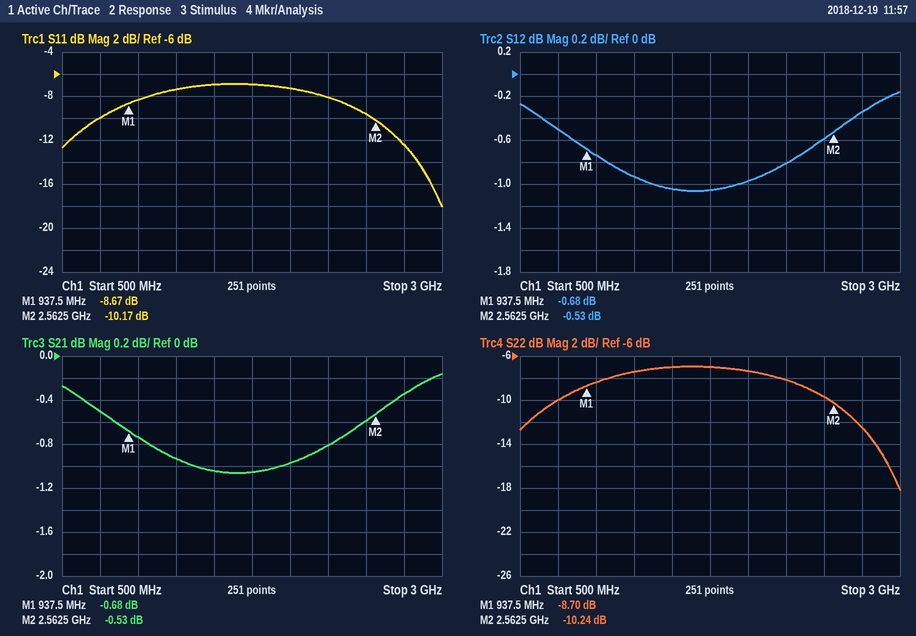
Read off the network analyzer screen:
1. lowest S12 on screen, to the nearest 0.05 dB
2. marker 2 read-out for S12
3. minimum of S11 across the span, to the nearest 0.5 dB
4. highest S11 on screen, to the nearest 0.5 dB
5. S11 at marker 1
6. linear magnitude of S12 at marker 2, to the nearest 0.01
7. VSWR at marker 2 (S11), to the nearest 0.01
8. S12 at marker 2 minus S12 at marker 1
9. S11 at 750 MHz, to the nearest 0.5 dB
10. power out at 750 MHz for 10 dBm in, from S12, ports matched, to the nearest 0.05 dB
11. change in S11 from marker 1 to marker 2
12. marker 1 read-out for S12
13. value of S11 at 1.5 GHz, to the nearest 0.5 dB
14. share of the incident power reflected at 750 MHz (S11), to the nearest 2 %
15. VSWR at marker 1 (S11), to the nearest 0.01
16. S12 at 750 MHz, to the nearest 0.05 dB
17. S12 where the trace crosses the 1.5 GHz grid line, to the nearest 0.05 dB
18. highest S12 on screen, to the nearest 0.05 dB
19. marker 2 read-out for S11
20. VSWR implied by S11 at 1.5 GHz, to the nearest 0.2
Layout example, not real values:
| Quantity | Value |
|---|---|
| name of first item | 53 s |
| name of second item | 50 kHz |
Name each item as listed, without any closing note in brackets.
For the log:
| Quantity | Value |
|---|---|
| lowest S12 on screen, to the nearest 0.05 dB | -1.05 dB |
| marker 2 read-out for S12 | -0.53 dB |
| minimum of S11 across the span, to the nearest 0.5 dB | -18.0 dB |
| highest S11 on screen, to the nearest 0.5 dB | -7.0 dB |
| S11 at marker 1 | -8.67 dB |
| linear magnitude of S12 at marker 2, to the nearest 0.01 | 0.94 |
| VSWR at marker 2 (S11), to the nearest 0.01 | 1.90 |
| S12 at marker 2 minus S12 at marker 1 | 0.15 dB |
| S11 at 750 MHz, to the nearest 0.5 dB | -10.0 dB |
| power out at 750 MHz for 10 dBm in, from S12, ports matched, to the nearest 0.05 dB | 9.50 dBm |
| change in S11 from marker 1 to marker 2 | -1.50 dB |
| marker 1 read-out for S12 | -0.68 dB |
| value of S11 at 1.5 GHz, to the nearest 0.5 dB | -7.0 dB |
| share of the incident power reflected at 750 MHz (S11), to the nearest 2 % | 10 % |
| VSWR at marker 1 (S11), to the nearest 0.01 | 2.17 |
| S12 at 750 MHz, to the nearest 0.05 dB | -0.50 dB |
| S12 where the trace crosses the 1.5 GHz grid line, to the nearest 0.05 dB | -1.05 dB |
| highest S12 on screen, to the nearest 0.05 dB | -0.15 dB |
| marker 2 read-out for S11 | -10.17 dB |
| VSWR implied by S11 at 1.5 GHz, to the nearest 0.2 | 2.6 |
